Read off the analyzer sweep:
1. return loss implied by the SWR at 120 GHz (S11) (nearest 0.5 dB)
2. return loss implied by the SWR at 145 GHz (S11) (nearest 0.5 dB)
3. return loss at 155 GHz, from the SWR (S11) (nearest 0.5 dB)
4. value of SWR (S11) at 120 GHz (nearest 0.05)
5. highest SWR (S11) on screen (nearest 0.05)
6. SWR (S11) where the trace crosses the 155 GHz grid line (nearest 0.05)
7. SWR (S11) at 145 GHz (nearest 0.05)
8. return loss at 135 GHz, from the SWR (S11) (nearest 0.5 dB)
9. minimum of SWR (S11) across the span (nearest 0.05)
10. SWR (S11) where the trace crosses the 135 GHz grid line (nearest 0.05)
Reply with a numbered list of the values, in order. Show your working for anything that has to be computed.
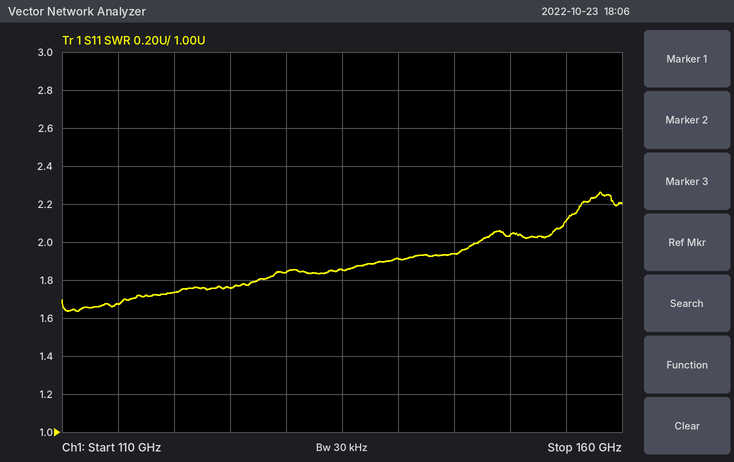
1. −20 log10((1.75 − 1)/(1.75 + 1)) ≈ 11.3 dB, so 11.5 dB to the nearest 0.5 dB
2. −20 log10((1.95 − 1)/(1.95 + 1)) ≈ 9.84 dB, so 10.0 dB to the nearest 0.5 dB
3. −20 log10((2.1 − 1)/(2.1 + 1)) ≈ 9.0 dB
4. 1.75
5. 2.25
6. 2.10
7. 1.95
8. −20 log10((1.85 − 1)/(1.85 + 1)) ≈ 10.5 dB
9. 1.65
10. 1.85
